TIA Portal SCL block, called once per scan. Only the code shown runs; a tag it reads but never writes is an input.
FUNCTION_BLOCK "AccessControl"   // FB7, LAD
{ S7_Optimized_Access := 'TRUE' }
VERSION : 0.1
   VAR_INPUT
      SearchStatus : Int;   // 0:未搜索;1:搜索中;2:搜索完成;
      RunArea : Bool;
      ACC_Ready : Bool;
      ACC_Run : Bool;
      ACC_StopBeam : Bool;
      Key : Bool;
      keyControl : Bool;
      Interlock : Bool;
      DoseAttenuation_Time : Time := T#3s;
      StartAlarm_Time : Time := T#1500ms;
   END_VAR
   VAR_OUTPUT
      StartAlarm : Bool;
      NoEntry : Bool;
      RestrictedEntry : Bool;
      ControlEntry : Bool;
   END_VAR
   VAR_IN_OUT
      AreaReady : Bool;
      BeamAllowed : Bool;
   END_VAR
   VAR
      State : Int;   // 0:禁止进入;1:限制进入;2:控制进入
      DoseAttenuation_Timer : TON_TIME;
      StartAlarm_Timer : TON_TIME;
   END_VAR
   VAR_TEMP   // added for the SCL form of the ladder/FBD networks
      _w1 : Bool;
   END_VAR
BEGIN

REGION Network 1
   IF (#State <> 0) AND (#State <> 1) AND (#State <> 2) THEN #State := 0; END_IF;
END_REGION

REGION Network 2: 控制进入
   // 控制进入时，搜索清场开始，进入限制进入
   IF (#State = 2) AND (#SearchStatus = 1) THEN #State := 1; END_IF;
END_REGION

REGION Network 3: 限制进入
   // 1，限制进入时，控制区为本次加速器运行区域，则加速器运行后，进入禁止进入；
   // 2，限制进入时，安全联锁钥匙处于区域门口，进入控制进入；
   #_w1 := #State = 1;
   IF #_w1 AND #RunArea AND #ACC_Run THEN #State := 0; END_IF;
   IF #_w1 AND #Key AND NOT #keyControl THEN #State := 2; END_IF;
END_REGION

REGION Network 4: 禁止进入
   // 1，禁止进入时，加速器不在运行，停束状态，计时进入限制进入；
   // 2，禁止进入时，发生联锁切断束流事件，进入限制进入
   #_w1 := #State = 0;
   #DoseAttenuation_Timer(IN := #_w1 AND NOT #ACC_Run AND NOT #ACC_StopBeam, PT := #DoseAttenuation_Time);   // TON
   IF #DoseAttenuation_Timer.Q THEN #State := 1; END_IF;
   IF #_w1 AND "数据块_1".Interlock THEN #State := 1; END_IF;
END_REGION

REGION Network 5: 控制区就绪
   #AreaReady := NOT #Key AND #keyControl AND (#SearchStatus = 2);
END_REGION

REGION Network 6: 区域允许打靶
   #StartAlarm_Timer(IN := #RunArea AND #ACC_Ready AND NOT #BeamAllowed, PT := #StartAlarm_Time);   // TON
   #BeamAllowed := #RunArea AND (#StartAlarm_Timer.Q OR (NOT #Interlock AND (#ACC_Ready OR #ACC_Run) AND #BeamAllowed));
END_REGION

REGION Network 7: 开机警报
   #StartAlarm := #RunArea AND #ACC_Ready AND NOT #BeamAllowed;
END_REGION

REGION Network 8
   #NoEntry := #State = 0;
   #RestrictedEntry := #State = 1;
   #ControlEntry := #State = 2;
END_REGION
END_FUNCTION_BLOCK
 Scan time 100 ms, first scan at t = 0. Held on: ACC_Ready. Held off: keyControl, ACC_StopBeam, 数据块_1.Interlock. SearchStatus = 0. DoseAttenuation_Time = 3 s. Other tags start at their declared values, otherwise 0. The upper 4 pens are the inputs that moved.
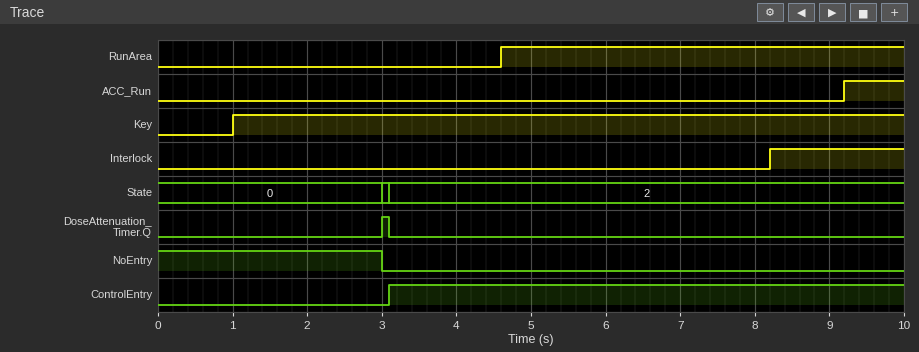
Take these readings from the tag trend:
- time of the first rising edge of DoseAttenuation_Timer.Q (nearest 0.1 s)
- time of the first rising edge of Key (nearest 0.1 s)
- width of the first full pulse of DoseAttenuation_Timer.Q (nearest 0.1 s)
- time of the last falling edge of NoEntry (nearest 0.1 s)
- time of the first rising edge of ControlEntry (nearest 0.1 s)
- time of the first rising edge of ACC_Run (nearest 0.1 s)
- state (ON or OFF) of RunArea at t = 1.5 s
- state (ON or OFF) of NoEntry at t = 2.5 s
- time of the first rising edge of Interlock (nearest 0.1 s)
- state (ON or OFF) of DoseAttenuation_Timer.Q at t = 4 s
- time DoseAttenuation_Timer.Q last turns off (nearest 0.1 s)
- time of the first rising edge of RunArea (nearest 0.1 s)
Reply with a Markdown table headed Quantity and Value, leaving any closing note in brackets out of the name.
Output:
| Quantity | Value |
|---|---|
| time of the first rising edge of DoseAttenuation_Timer.Q | 3.0 s |
| time of the first rising edge of Key | 1.0 s |
| width of the first full pulse of DoseAttenuation_Timer.Q | 0.1 s |
| time of the last falling edge of NoEntry | 3.0 s |
| time of the first rising edge of ControlEntry | 3.1 s |
| time of the first rising edge of ACC_Run | 9.2 s |
| state (ON or OFF) of RunArea at t = 1.5 s | OFF |
| state (ON or OFF) of NoEntry at t = 2.5 s | ON |
| time of the first rising edge of Interlock | 8.2 s |
| state (ON or OFF) of DoseAttenuation_Timer.Q at t = 4 s | OFF |
| time DoseAttenuation_Timer.Q last turns off | 3.1 s |
| time of the first rising edge of RunArea | 4.6 s |
